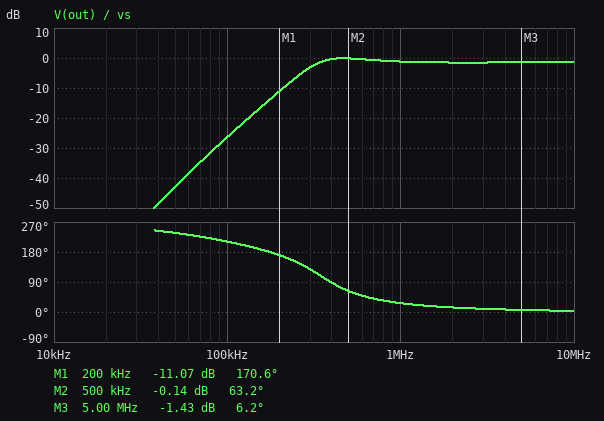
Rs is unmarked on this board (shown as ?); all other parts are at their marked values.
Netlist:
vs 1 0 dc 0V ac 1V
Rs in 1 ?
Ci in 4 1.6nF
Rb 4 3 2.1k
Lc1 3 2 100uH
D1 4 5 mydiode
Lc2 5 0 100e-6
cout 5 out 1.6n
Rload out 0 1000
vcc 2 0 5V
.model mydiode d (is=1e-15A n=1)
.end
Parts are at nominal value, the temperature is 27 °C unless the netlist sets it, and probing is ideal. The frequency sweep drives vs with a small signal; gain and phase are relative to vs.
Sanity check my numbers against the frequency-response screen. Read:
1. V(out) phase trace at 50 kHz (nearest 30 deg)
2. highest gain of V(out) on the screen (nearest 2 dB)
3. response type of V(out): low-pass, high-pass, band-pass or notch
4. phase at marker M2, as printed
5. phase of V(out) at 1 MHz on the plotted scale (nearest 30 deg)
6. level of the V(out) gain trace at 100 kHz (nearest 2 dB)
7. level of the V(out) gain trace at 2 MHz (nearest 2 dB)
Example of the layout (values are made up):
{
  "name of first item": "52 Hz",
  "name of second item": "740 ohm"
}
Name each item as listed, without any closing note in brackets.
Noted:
{
  "V(out) phase trace at 50 kHz": "240 deg",
  "highest gain of V(out) on the screen": "0 dB",
  "response type of V(out): low-pass, high-pass, band-pass or notch": "high-pass",
  "phase at marker M2, as printed": "63.2 deg",
  "phase of V(out) at 1 MHz on the plotted scale": "30 deg",
  "level of the V(out) gain trace at 100 kHz": "-26 dB",
  "level of the V(out) gain trace at 2 MHz": "-2 dB"
}
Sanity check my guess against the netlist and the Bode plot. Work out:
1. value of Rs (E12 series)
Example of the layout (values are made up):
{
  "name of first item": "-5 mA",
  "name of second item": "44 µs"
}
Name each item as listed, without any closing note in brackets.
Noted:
{
  "value of Rs": "150 Ω"
}
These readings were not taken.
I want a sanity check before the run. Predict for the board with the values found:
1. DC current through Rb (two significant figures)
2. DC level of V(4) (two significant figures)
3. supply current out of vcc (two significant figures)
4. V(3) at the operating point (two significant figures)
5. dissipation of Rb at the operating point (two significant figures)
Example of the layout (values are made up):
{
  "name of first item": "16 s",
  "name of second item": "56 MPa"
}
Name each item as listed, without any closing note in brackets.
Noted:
{
  "DC current through Rb": "2.0 mA",
  "DC level of V(4)": "730 mV",
  "supply current out of vcc": "2.0 mA",
  "V(3) at the operating point": "5.0 V",
  "dissipation of Rb at the operating point": "8.7 mW"
}
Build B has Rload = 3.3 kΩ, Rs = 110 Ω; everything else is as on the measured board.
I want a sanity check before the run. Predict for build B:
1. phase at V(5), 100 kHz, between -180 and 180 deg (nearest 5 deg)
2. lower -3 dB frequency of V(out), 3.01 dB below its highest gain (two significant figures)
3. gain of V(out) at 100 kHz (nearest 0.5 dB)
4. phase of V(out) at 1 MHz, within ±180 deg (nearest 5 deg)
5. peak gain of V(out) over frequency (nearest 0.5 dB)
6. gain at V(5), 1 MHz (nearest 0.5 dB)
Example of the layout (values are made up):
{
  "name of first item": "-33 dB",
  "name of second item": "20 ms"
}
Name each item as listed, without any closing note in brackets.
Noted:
{
  "phase at V(5), 100 kHz, between -180 and 180 deg": "170 deg",
  "lower -3 dB frequency of V(out), 3.01 dB below its highest gain": "320 kHz",
  "gain of V(out) at 100 kHz": "-24.0 dB",
  "phase of V(out) at 1 MHz, within ±180 deg": "20 deg",
  "peak gain of V(out) over frequency": "3.5 dB",
  "gain at V(5), 1 MHz": "0.5 dB"
}
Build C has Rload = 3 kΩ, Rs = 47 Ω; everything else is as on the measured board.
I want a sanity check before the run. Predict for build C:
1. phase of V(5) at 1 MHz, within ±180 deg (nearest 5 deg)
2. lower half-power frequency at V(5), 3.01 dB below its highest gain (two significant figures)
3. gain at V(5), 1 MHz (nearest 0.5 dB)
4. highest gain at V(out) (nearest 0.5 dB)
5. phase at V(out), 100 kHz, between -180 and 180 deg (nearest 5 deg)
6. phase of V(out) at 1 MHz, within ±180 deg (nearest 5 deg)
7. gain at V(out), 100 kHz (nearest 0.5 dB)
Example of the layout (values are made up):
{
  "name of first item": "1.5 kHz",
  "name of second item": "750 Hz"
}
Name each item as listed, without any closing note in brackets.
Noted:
{
  "phase of V(5) at 1 MHz, within ±180 deg": "10 deg",
  "lower half-power frequency at V(5), 3.01 dB below its highest gain": "340 kHz",
  "gain at V(5), 1 MHz": "1.0 dB",
  "highest gain at V(out)": "7.0 dB",
  "phase at V(out), 100 kHz, between -180 and 180 deg": "-170 deg",
  "phase of V(out) at 1 MHz, within ±180 deg": "15 deg",
  "gain at V(out), 100 kHz": "-24.0 dB"
}
